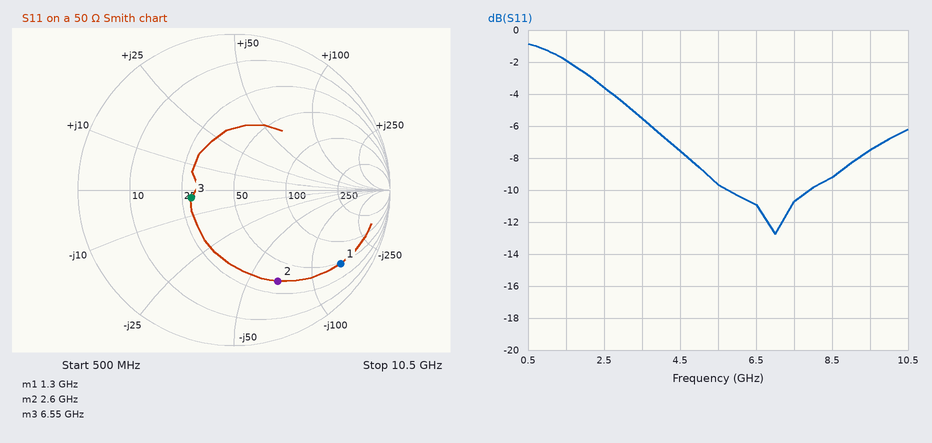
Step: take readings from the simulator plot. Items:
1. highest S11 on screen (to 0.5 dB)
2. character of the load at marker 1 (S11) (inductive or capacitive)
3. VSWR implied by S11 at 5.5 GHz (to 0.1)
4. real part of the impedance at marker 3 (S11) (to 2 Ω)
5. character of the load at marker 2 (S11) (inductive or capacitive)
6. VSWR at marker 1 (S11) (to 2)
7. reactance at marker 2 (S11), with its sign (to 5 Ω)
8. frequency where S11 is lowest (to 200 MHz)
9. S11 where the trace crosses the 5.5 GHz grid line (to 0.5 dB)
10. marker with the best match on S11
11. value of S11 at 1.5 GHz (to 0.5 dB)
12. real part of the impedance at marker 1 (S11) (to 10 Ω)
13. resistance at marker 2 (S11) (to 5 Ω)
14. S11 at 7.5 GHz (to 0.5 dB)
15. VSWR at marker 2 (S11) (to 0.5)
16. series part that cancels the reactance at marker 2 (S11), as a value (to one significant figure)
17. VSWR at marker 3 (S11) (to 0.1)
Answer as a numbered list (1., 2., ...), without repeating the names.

1. -1.0 dB
2. capacitive
3. 2.0
4. 28 Ω
5. capacitive
6. 10
7. -70 Ω
8. 7.0 GHz
9. -9.5 dB
10. marker 3
11. -2.0 dB
12. 50 Ω
13. 35 Ω
14. -10.5 dB
15. 4.5
16. 4 nH
17. 1.8
